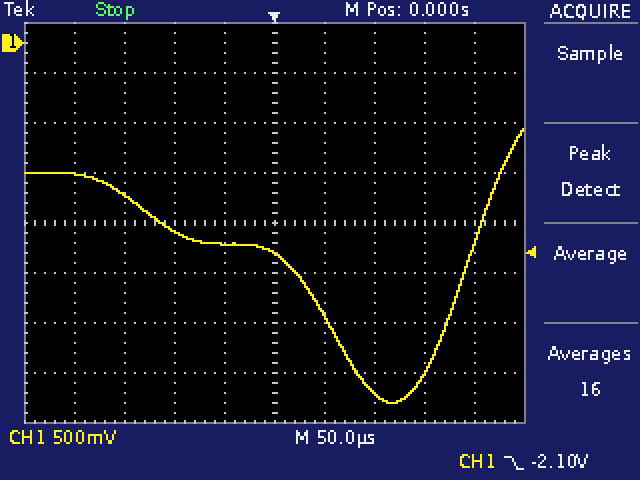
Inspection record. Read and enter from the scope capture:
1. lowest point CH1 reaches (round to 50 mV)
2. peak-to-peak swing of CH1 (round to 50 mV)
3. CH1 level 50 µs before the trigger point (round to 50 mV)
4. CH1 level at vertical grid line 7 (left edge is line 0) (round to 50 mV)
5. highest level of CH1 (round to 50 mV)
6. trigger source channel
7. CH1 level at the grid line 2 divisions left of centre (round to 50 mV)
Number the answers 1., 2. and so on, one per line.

1. -3.60 V
2. 2.75 V
3. -2.00 V
4. -3.50 V
5. -850 mV
6. CH1
7. -1.90 V
